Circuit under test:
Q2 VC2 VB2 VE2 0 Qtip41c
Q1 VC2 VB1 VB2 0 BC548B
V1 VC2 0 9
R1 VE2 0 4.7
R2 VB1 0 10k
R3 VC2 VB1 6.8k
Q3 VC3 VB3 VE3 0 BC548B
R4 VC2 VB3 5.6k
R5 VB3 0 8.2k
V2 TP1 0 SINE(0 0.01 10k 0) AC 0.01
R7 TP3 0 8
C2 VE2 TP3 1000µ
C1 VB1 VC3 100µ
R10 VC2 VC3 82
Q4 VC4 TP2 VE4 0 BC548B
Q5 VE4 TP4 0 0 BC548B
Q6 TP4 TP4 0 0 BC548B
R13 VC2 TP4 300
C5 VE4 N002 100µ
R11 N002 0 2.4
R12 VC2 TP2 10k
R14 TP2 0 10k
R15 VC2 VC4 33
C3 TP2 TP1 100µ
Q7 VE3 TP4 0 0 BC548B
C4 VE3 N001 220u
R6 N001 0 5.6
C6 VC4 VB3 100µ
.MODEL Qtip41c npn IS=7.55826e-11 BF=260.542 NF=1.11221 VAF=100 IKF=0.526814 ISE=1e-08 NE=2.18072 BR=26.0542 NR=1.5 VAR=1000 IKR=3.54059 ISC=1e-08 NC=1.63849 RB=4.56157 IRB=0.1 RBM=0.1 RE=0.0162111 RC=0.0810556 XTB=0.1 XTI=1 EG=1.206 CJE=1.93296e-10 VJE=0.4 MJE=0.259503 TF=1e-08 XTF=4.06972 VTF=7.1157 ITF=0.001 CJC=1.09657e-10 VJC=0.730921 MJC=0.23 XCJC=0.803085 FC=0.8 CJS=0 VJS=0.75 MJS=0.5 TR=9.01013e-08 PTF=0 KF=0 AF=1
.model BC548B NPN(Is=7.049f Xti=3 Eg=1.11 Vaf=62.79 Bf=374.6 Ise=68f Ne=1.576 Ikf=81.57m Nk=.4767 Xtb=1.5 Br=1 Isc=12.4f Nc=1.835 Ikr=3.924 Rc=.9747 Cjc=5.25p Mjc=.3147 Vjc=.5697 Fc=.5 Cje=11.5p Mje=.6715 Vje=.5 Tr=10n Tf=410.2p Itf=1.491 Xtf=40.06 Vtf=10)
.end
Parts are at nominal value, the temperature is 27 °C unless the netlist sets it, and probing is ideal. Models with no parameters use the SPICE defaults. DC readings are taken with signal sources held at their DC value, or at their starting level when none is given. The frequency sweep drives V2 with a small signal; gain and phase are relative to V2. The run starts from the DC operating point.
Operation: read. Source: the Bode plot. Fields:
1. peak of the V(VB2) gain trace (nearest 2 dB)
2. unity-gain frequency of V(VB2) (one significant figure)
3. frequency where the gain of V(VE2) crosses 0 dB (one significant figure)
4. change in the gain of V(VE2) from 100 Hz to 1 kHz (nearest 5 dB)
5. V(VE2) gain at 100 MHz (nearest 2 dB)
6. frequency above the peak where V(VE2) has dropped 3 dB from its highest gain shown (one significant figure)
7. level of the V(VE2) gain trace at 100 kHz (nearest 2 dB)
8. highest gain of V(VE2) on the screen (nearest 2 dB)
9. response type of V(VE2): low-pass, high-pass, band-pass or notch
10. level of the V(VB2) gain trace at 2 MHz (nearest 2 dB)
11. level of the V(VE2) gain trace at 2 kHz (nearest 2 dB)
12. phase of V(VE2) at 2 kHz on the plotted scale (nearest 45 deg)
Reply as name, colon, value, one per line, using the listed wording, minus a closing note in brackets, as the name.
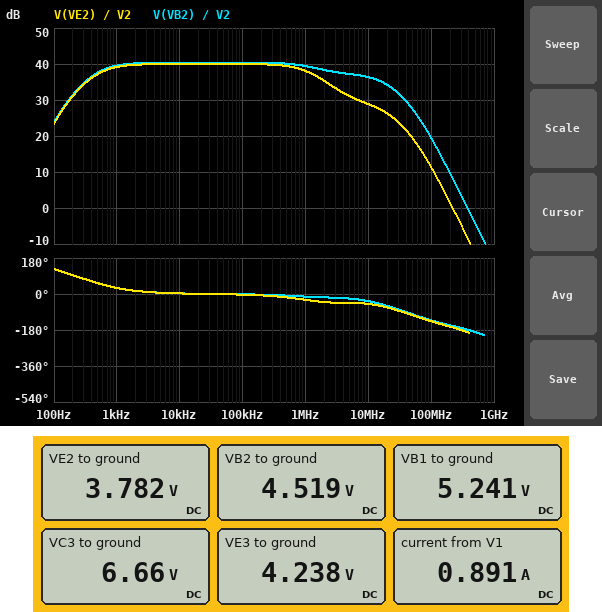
peak of the V(VB2) gain trace: 40 dB
unity-gain frequency of V(VB2): 400 MHz
frequency where the gain of V(VE2) crosses 0 dB: 200 MHz
change in the gain of V(VE2) from 100 Hz to 1 kHz: 15 dB
V(VE2) gain at 100 MHz: 12 dB
frequency above the peak where V(VE2) has dropped 3 dB from its highest gain shown: 1 MHz
level of the V(VE2) gain trace at 100 kHz: 40 dB
highest gain of V(VE2) on the screen: 40 dB
response type of V(VE2): low-pass, high-pass, band-pass or notch: band-pass
level of the V(VB2) gain trace at 2 MHz: 38 dB
level of the V(VE2) gain trace at 2 kHz: 40 dB
phase of V(VE2) at 2 kHz on the plotted scale: 0 deg
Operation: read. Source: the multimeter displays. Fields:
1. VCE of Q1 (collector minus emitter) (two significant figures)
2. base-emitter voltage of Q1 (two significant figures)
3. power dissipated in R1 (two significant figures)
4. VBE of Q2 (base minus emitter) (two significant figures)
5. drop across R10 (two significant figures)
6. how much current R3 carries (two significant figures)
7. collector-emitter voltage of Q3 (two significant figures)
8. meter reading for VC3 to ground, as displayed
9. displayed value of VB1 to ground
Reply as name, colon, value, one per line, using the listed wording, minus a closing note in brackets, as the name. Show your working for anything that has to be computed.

VCE of Q1 (collector minus emitter): 9 V - 4.519 V = 4.5 V
base-emitter voltage of Q1: 5.241 V - 4.519 V = 720 mV
power dissipated in R1: (3.782 V)^2 / 4.7 Ω = 3.0 W
VBE of Q2 (base minus emitter): 4.519 V - 3.782 V = 740 mV
drop across R10: 9 V - 6.66 V = 2.3 V
how much current R3 carries: (9 V - 5.241 V) / 6.8 kΩ = 550 µA
collector-emitter voltage of Q3: 6.66 V - 4.238 V = 2.4 V
meter reading for VC3 to ground, as displayed: 6.66 V
displayed value of VB1 to ground: 5.241 V
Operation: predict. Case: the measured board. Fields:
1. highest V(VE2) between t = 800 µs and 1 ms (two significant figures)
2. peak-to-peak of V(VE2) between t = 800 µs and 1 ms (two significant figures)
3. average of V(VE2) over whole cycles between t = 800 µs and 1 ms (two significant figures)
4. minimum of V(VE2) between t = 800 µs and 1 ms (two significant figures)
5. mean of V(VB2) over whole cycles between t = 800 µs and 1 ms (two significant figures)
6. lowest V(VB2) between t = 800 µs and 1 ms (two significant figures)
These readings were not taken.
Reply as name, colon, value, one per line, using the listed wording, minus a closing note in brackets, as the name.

highest V(VE2) between t = 800 µs and 1 ms: 4.8 V
peak-to-peak of V(VE2) between t = 800 µs and 1 ms: 2.0 V
average of V(VE2) over whole cycles between t = 800 µs and 1 ms: 3.8 V
minimum of V(VE2) between t = 800 µs and 1 ms: 2.8 V
mean of V(VB2) over whole cycles between t = 800 µs and 1 ms: 4.5 V
lowest V(VB2) between t = 800 µs and 1 ms: 3.5 V
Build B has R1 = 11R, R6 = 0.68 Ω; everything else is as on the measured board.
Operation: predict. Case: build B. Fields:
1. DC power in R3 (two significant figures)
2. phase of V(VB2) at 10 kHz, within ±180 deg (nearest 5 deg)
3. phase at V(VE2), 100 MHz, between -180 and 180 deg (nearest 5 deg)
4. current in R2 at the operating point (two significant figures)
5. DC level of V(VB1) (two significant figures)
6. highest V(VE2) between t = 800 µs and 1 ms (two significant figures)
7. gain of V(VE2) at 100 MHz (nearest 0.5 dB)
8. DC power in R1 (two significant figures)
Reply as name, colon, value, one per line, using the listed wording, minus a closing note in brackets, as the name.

DC power in R3: 2.0 mW
phase of V(VB2) at 10 kHz, within ±180 deg: 5 deg
phase at V(VE2), 100 MHz, between -180 and 180 deg: -145 deg
current in R2 at the operating point: 530 µA
DC level of V(VB1): 5.3 V
highest V(VE2) between t = 800 µs and 1 ms: 6.0 V
gain of V(VE2) at 100 MHz: 15.0 dB
DC power in R1: 1.4 W
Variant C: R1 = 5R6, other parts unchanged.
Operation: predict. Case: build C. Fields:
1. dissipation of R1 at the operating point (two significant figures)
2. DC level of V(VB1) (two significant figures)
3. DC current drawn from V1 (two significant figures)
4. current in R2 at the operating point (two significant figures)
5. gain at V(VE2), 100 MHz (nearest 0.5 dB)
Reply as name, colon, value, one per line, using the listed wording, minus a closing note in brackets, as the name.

dissipation of R1 at the operating point: 2.6 W
DC level of V(VB1): 5.3 V
DC current drawn from V1: 770 mA
current in R2 at the operating point: 530 µA
gain at V(VE2), 100 MHz: 12.0 dB
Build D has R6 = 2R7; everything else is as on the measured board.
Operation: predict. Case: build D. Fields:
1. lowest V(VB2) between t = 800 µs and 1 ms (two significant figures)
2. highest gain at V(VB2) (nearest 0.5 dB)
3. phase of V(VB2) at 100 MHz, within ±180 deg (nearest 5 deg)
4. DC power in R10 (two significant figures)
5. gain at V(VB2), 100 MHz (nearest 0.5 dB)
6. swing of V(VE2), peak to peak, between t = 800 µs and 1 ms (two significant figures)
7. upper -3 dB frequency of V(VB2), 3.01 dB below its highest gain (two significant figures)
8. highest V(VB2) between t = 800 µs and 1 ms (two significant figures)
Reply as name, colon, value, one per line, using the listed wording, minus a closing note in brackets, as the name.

lowest V(VB2) between t = 800 µs and 1 ms: 2.7 V
highest gain at V(VB2): 45.0 dB
phase of V(VB2) at 100 MHz, within ±180 deg: -140 deg
DC power in R10: 67 mW
gain at V(VB2), 100 MHz: 21.0 dB
swing of V(VE2), peak to peak, between t = 800 µs and 1 ms: 3.3 V
upper -3 dB frequency of V(VB2), 3.01 dB below its highest gain: 3.9 MHz
highest V(VB2) between t = 800 µs and 1 ms: 6.1 V
